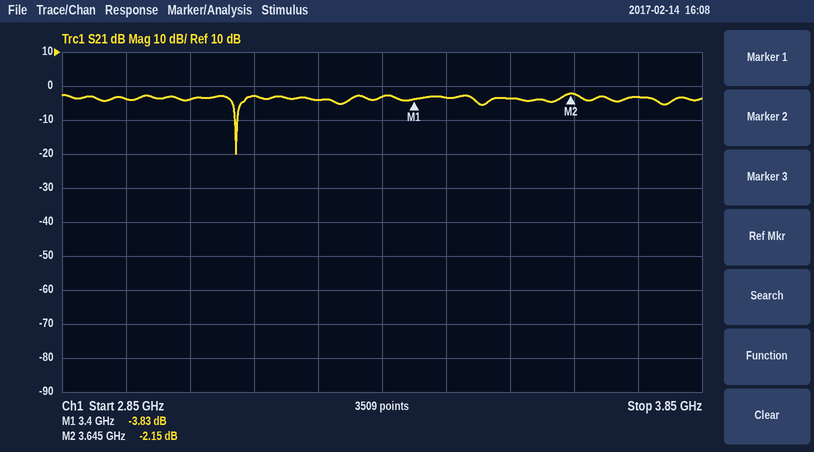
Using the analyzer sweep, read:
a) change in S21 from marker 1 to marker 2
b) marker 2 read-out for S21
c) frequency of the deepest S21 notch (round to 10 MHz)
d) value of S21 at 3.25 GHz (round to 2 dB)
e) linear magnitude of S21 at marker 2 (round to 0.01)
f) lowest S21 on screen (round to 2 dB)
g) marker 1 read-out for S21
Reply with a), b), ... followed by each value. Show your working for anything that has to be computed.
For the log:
a) -2.15 − (-3.83) = 1.68 dB
b) -2.15 dB
c) 3.12 GHz
d) -4 dB
e) 10^(-2.15/20) ≈ 0.78
f) -20 dB
g) -3.83 dB
